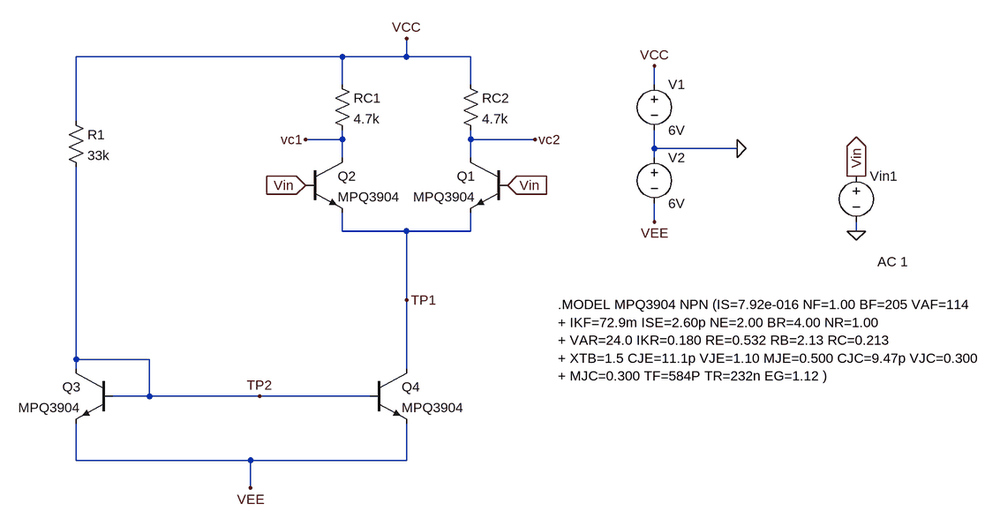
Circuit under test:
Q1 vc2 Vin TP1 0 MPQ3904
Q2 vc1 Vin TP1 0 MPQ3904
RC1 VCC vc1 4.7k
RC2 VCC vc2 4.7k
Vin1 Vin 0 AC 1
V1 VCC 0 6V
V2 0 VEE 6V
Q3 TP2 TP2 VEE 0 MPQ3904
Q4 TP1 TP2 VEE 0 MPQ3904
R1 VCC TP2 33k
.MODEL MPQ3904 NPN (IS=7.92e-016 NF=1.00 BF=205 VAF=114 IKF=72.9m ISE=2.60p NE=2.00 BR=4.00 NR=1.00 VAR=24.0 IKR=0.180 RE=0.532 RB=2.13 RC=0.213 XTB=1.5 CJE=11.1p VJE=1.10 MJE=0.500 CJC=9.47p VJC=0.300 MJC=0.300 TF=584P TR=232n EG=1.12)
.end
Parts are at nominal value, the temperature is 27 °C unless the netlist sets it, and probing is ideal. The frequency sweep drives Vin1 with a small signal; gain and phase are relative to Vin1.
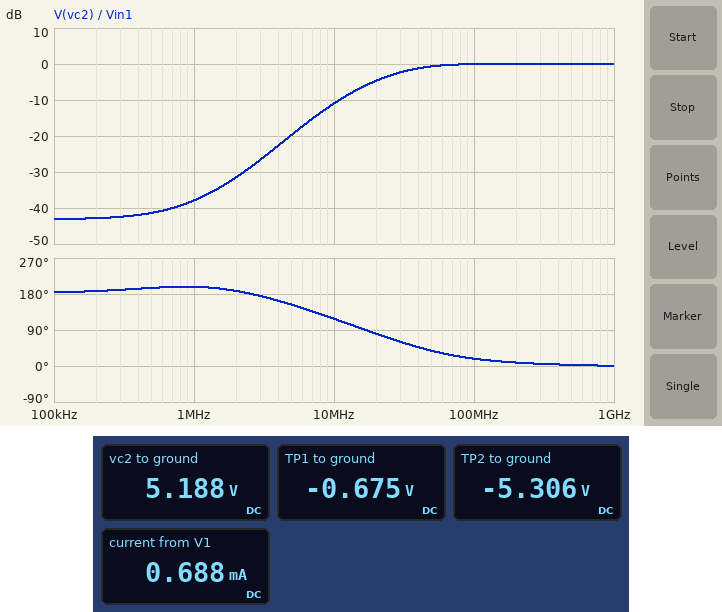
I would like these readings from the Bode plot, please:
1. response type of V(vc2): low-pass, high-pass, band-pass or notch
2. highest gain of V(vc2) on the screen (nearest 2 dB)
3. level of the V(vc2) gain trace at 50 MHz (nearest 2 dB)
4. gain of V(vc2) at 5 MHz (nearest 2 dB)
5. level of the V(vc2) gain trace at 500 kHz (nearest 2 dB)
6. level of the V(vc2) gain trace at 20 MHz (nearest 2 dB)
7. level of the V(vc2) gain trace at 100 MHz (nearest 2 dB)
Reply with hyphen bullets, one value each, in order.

- high-pass
- 0 dB
- 0 dB
- -20 dB
- -42 dB
- -4 dB
- 0 dB
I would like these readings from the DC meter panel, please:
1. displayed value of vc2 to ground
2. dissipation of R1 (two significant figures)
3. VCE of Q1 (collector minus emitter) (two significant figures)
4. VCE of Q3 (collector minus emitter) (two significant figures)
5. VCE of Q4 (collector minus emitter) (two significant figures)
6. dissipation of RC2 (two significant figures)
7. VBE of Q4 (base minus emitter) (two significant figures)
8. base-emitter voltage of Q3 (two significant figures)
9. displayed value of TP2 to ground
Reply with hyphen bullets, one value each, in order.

- 5.188 V
- 3.9 mW
- 5.9 V
- 690 mV
- 5.3 V
- 140 µW
- 690 mV
- 690 mV
- -5.306 V
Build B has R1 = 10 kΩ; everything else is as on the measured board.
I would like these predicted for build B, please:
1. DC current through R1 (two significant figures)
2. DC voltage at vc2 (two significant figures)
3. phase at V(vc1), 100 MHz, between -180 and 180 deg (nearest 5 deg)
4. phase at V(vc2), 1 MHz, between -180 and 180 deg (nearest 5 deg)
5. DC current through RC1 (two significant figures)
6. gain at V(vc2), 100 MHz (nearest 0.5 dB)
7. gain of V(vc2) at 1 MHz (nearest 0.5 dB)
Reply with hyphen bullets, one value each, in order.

- 1.1 mA
- 3.3 V
- 35 deg
- 160 deg
- 570 µA
- -1.0 dB
- -32.0 dB
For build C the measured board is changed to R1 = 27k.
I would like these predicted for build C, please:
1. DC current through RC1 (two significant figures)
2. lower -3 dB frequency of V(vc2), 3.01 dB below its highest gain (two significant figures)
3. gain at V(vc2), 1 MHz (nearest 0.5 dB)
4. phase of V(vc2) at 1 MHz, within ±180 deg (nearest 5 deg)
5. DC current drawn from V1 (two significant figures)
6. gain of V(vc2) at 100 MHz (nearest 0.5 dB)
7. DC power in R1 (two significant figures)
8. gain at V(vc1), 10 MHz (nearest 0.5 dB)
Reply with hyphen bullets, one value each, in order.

- 210 µA
- 30 MHz
- -37.5 dB
- -165 deg
- 840 µA
- 0 dB
- 4.7 mW
- -12.0 dB
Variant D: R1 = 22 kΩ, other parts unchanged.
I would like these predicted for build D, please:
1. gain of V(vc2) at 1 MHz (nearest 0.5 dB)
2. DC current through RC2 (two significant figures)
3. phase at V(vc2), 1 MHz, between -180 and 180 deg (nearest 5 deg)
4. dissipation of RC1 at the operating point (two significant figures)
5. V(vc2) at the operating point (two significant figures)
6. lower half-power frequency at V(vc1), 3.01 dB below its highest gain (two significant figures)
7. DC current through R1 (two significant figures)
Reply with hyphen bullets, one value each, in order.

- -37.0 dB
- 260 µA
- -170 deg
- 320 µW
- 4.8 V
- 34 MHz
- 510 µA
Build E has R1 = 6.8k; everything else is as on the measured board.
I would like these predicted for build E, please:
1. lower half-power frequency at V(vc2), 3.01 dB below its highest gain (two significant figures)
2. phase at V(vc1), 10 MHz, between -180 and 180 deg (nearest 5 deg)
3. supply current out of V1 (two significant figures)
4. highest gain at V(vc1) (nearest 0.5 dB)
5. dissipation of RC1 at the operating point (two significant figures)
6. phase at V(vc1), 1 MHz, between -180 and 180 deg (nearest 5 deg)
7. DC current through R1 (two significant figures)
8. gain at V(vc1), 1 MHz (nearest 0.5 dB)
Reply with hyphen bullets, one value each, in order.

- 66 MHz
- 75 deg
- 3.3 mA
- 0 dB
- 3.3 mW
- 140 deg
- 1.7 mA
- -28.0 dB
